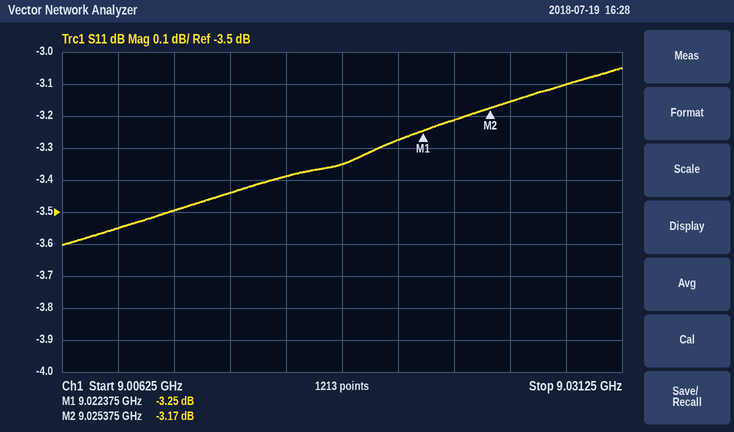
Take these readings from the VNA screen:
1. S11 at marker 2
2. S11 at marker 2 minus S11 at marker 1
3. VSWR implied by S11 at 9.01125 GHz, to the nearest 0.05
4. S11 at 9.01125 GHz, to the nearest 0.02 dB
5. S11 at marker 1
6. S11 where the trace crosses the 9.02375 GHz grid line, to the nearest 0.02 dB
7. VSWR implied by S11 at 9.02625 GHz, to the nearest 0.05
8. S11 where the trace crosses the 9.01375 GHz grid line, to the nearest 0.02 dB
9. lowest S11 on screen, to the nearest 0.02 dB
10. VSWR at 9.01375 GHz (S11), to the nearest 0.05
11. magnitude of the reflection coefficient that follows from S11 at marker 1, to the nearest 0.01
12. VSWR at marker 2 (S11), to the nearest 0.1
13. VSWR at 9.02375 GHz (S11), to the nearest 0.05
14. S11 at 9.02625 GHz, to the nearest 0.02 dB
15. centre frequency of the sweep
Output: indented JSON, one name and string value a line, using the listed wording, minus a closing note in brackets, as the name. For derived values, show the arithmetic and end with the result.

{
  "S11 at marker 2": "-3.17 dB",
  "S11 at marker 2 minus S11 at marker 1": "-3.17 − (-3.25) = 0.08 dB",
  "VSWR implied by S11 at 9.01125 GHz, to the nearest 0.05": "|Γ| = 10^(-3.5/20) = 0.6683; VSWR = (1 + 0.6683)/(1 − 0.6683) ≈ 5.03, so 5.05 to the nearest 0.05",
  "S11 at 9.01125 GHz, to the nearest 0.02 dB": "-3.50 dB",
  "S11 at marker 1": "-3.25 dB",
  "S11 where the trace crosses the 9.02375 GHz grid line, to the nearest 0.02 dB": "-3.22 dB",
  "VSWR implied by S11 at 9.02625 GHz, to the nearest 0.05": "|Γ| = 10^(-3.16/20) = 0.6950; VSWR = (1 + 0.6950)/(1 − 0.6950) ≈ 5.56, so 5.55 to the nearest 0.05",
  "S11 where the trace crosses the 9.01375 GHz grid line, to the nearest 0.02 dB": "-3.44 dB",
  "lowest S11 on screen, to the nearest 0.02 dB": "-3.60 dB",
  "VSWR at 9.01375 GHz (S11), to the nearest 0.05": "|Γ| = 10^(-3.44/20) = 0.6730; VSWR = (1 + 0.6730)/(1 − 0.6730) ≈ 5.12, so 5.10 to the nearest 0.05",
  "magnitude of the reflection coefficient that follows from S11 at marker 1, to the nearest 0.01": "10^(-3.25/20) ≈ 0.69",
  "VSWR at marker 2 (S11), to the nearest 0.1": "(1 + 0.6942)/(1 − 0.6942) ≈ 5.5",
  "VSWR at 9.02375 GHz (S11), to the nearest 0.05": "|Γ| = 10^(-3.22/20) = 0.6902; VSWR = (1 + 0.6902)/(1 − 0.6902) ≈ 5.46, so 5.45 to the nearest 0.05",
  "S11 at 9.02625 GHz, to the nearest 0.02 dB": "-3.16 dB",
  "centre frequency of the sweep": "9.01875 GHz"
}
